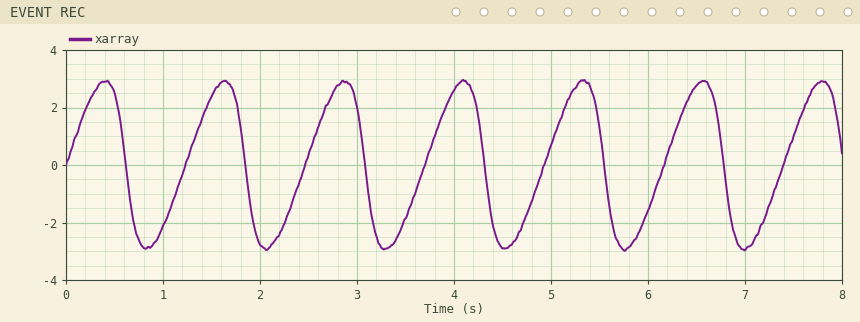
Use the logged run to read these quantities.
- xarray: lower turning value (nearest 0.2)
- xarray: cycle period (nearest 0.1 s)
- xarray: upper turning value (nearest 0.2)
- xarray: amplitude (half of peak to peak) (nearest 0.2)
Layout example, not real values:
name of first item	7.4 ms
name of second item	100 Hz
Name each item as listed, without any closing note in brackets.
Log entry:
xarray: lower turning value	-3.0
xarray: cycle period	1.2 s
xarray: upper turning value	3.0
xarray: amplitude (half of peak to peak)	3.0
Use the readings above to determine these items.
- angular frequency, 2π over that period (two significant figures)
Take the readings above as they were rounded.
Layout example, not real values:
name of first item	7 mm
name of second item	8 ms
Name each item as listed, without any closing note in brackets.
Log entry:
angular frequency, 2π over that period	5.2 rad/s
